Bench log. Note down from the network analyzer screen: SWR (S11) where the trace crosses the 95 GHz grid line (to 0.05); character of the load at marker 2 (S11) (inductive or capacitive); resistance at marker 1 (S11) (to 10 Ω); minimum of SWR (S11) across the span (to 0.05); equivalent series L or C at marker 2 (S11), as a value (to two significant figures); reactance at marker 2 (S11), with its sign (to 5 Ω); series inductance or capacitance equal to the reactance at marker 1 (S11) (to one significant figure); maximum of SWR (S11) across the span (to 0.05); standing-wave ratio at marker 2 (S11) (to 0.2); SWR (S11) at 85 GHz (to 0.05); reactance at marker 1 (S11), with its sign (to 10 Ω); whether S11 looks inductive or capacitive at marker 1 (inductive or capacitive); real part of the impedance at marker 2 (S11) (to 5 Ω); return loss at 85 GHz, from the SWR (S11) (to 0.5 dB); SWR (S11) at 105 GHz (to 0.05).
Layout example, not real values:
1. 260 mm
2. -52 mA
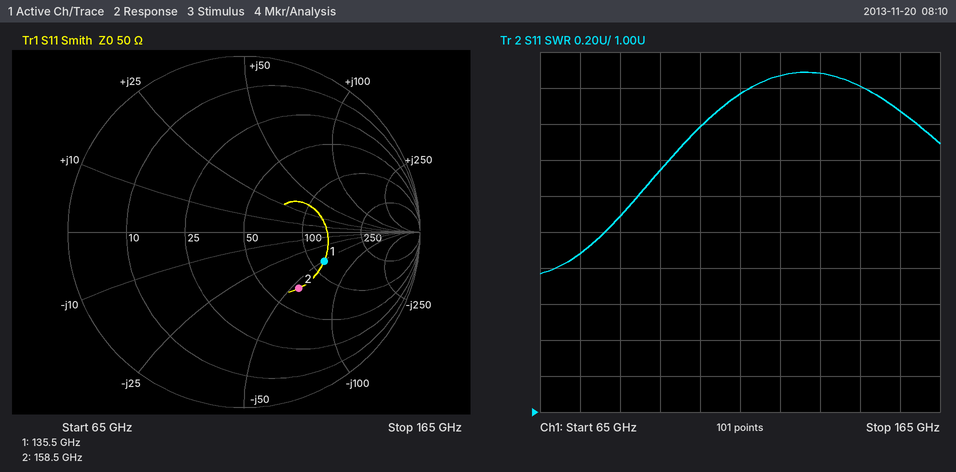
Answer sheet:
1. 2.35
2. capacitive
3. 120 Ω
4. 1.75
5. 18 fF
6. -55 Ω
7. 20 fF
8. 2.90
9. 2.6
10. 2.10
11. -50 Ω
12. capacitive
13. 70 Ω
14. 9.0 dB
15. 2.60
